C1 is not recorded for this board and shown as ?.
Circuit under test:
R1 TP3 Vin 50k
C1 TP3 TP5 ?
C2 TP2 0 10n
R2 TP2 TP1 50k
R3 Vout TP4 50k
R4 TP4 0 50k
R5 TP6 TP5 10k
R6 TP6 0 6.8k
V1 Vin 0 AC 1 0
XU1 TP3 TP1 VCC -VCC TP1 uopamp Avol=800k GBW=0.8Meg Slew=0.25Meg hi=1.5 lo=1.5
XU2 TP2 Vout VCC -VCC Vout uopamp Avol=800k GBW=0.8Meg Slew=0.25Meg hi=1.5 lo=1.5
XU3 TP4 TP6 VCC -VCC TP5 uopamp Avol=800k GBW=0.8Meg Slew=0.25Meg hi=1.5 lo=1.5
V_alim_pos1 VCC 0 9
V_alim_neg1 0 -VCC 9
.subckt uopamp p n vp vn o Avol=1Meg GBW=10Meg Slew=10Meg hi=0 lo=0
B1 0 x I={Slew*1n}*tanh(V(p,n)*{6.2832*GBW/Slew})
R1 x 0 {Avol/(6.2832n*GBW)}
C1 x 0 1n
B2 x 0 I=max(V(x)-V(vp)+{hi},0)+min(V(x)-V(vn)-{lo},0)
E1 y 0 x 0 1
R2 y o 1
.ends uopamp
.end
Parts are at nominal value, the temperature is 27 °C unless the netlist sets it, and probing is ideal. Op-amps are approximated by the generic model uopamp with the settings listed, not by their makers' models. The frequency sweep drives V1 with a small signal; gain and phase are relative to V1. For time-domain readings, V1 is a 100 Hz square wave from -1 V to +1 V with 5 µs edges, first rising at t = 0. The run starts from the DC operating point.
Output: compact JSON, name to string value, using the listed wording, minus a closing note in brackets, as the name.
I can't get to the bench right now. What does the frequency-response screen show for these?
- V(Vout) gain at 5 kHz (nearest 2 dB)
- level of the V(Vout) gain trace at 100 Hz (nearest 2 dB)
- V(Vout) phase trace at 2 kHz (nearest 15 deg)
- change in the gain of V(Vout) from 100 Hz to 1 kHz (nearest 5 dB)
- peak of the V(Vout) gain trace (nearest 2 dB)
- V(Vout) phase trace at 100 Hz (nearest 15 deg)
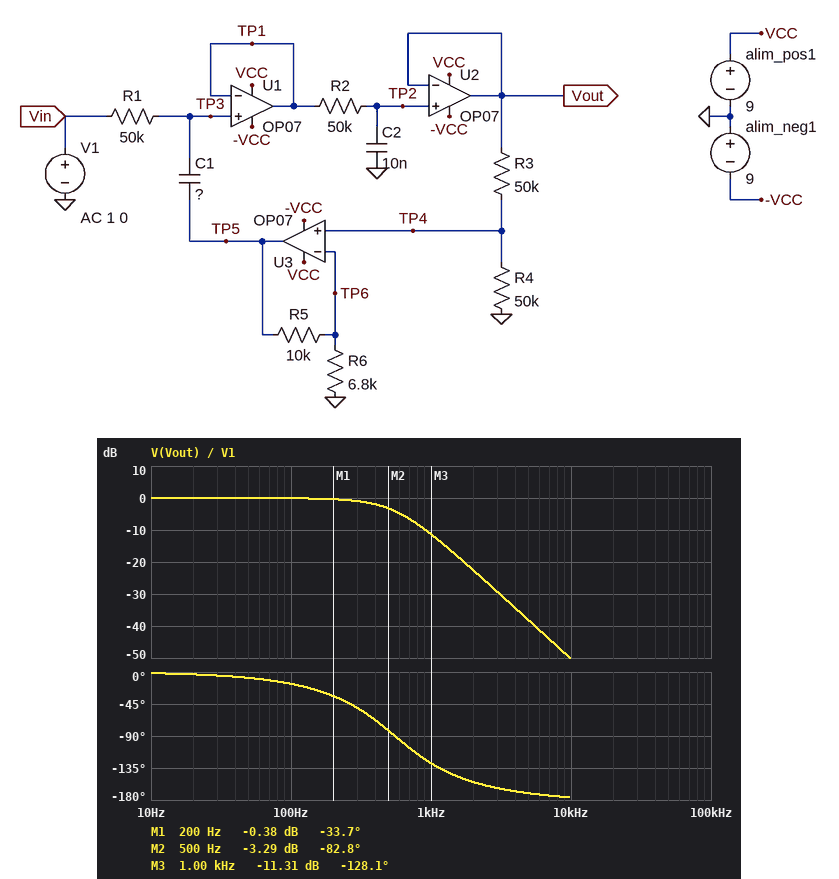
{"V(Vout) gain at 5 kHz": "-38 dB", "level of the V(Vout) gain trace at 100 Hz": "0 dB", "V(Vout) phase trace at 2 kHz": "-150 deg", "change in the gain of V(Vout) from 100 Hz to 1 kHz": "-10 dB", "peak of the V(Vout) gain trace": "0 dB", "V(Vout) phase trace at 100 Hz": "-15 deg"}
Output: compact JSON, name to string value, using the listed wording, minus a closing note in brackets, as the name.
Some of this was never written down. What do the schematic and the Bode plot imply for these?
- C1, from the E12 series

{"C1, from the E12 series": "3.3 nF"}
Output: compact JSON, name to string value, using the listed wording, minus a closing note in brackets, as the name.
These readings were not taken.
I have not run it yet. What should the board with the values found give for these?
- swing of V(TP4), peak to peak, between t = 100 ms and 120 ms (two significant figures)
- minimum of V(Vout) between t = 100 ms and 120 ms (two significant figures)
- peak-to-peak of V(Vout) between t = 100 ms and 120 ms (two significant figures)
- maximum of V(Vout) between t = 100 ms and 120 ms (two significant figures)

{"swing of V(TP4), peak to peak, between t = 100 ms and 120 ms": "1.0 V", "minimum of V(Vout) between t = 100 ms and 120 ms": "-1.0 V", "peak-to-peak of V(Vout) between t = 100 ms and 120 ms": "2.1 V", "maximum of V(Vout) between t = 100 ms and 120 ms": "1.0 V"}
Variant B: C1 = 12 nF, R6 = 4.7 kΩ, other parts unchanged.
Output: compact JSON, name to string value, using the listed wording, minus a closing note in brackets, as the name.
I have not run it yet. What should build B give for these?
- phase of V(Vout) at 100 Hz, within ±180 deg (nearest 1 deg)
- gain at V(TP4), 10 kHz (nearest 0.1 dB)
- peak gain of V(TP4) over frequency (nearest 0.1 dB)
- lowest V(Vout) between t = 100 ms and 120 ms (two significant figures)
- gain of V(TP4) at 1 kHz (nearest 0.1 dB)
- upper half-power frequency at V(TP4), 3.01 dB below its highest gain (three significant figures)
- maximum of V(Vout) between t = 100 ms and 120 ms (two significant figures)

{"phase of V(Vout) at 100 Hz, within ±180 deg": "-7 deg", "gain at V(TP4), 10 kHz": "-67.5 dB", "peak gain of V(TP4) over frequency": "4.7 dB", "lowest V(Vout) between t = 100 ms and 120 ms": "-2.6 V", "gain of V(TP4) at 1 kHz": "-26.8 dB", "upper half-power frequency at V(TP4), 3.01 dB below its highest gain": "324 Hz", "maximum of V(Vout) between t = 100 ms and 120 ms": "2.6 V"}
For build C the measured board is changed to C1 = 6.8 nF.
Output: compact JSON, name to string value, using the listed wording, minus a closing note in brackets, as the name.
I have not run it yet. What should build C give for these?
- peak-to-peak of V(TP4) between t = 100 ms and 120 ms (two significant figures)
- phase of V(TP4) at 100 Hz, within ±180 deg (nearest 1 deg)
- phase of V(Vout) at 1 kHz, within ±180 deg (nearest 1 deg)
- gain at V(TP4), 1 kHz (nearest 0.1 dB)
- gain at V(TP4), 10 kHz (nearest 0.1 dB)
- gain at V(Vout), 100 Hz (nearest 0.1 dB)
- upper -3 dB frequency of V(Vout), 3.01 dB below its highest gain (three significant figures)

{"peak-to-peak of V(TP4) between t = 100 ms and 120 ms": "1.3 V", "phase of V(TP4) at 100 Hz, within ±180 deg": "-16 deg", "phase of V(Vout) at 1 kHz, within ±180 deg": "-155 deg", "gain at V(TP4), 1 kHz": "-22.0 dB", "gain at V(TP4), 10 kHz": "-62.6 dB", "gain at V(Vout), 100 Hz": "0.3 dB", "upper -3 dB frequency of V(Vout), 3.01 dB below its highest gain": "449 Hz"}
